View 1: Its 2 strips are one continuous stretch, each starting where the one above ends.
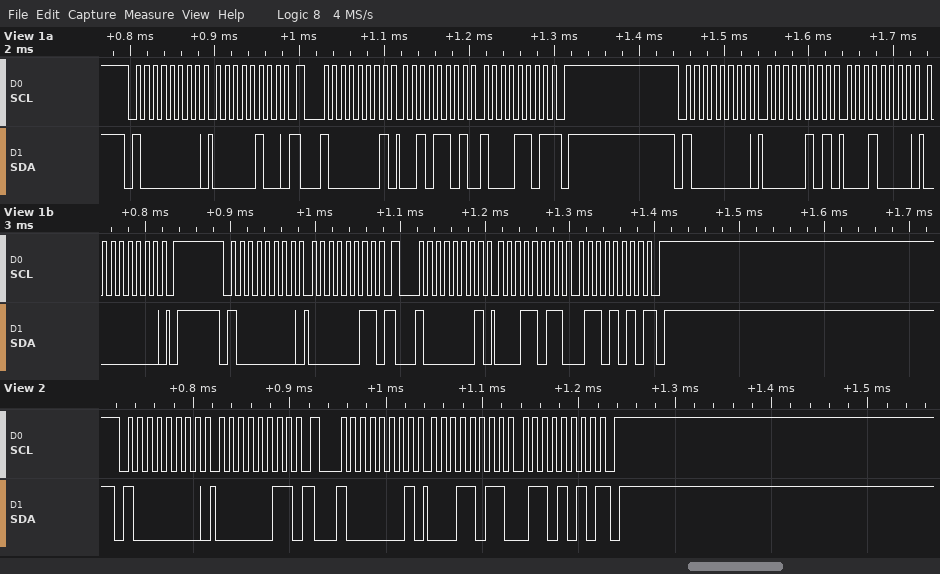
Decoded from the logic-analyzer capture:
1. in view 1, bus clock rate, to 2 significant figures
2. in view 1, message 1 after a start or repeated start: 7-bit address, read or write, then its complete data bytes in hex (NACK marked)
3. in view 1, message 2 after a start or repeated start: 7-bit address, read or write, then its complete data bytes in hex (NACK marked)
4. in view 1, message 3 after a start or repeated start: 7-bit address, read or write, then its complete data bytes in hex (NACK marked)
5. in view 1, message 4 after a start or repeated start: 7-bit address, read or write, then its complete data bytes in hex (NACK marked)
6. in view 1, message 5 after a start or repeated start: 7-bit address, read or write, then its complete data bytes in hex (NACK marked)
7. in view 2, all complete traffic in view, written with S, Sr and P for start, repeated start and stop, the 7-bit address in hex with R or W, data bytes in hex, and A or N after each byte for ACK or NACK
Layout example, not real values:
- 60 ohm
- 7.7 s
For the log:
- 100 kHz
- 0x40 write: 04
- 0x40 read: 2D 8D NACK
- 0x40 write: 05 10 00
- 0x40 write: 03
- 0x40 read: 1B 6A NACK
- S 40W A 03 A Sr 40R A 1B A 6A N P
